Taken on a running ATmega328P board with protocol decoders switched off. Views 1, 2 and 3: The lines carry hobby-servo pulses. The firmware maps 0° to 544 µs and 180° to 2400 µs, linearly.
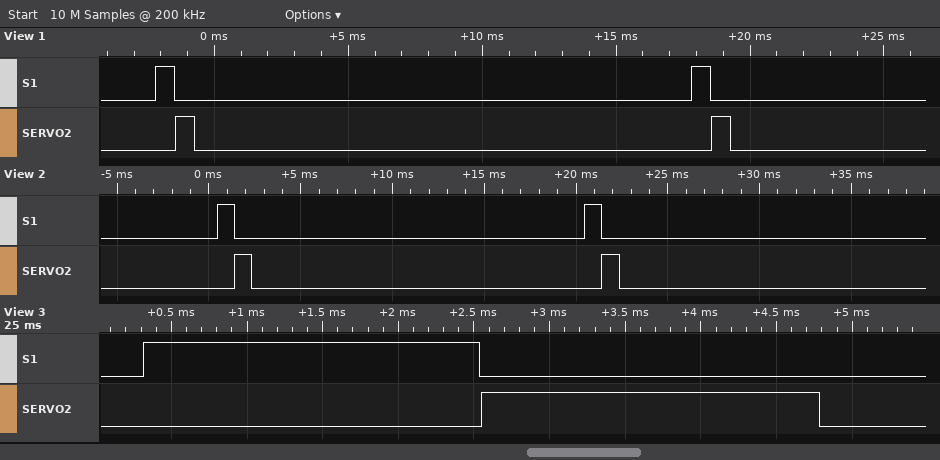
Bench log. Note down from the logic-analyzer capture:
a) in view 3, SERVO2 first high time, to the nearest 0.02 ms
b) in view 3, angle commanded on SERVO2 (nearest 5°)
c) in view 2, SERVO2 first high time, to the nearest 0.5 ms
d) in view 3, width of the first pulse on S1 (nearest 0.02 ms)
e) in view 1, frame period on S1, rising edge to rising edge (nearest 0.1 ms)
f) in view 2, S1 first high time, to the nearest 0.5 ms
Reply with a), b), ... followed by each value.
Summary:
a) 2.24 ms
b) 165°
c) 1.0 ms
d) 2.22 ms
e) 20.0 ms
f) 1.0 ms
